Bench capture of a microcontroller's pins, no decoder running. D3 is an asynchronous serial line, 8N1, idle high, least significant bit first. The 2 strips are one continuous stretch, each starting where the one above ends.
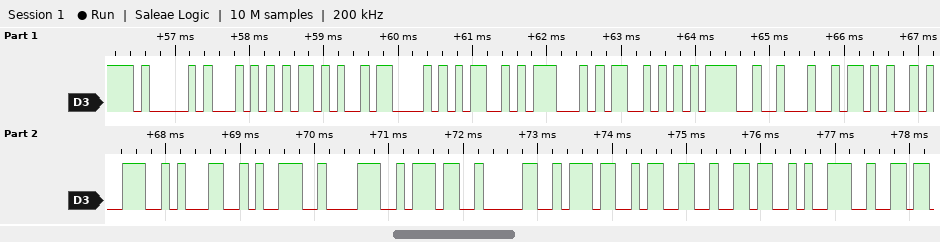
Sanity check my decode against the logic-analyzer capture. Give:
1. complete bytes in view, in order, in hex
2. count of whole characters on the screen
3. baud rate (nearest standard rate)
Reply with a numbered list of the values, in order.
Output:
1. 0x41 0x54 0x2B 0x43 0x4D 0x47 0x53 0x3D 0x22 0x2B 0x39 0x31 0x39 0x38 0x37 0x30 0x37 0x33 0x36 0x39
2. 20
3. 9600 baud
